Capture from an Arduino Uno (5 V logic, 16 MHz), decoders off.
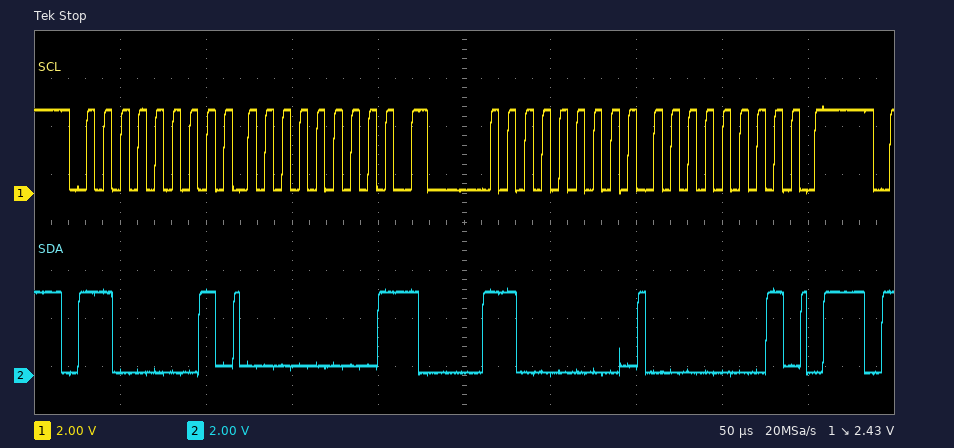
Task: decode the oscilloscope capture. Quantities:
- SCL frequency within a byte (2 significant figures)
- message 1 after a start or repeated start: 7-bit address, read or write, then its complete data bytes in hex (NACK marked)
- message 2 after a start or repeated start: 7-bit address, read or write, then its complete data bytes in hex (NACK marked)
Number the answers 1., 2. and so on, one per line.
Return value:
1. 100 kHz
2. 0x60 read: 00 NACK
3. 0x60 write: 01
